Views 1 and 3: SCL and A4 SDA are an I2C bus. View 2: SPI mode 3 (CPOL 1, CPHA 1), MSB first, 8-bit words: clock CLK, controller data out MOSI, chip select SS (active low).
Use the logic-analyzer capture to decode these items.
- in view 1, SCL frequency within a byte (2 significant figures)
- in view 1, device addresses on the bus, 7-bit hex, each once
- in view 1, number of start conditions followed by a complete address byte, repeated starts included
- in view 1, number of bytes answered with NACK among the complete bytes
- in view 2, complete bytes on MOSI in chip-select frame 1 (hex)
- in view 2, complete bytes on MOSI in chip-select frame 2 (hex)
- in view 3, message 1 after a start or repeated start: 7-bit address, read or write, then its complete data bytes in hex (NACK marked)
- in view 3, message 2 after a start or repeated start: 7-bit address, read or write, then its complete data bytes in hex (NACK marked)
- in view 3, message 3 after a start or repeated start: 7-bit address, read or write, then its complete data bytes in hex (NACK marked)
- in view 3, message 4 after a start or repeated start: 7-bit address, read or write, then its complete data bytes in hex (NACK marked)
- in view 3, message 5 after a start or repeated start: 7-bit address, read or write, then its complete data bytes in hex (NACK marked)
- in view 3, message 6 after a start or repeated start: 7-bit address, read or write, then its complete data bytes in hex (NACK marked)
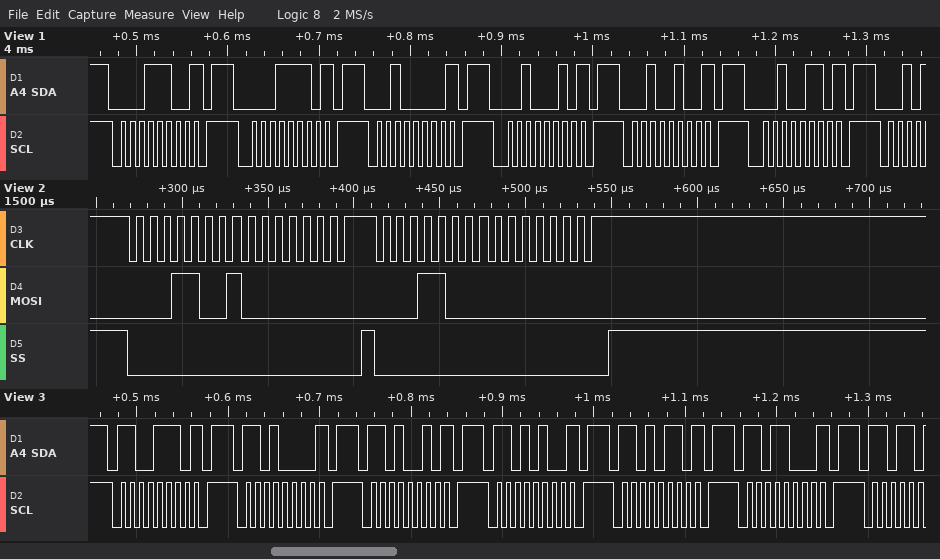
100 kHz
0x0E 0x0F 0x10 0x11 0x12 0x13
6
6
19 00
18 00
0x67 write NACK
0x68 write NACK
0x69 write NACK
0x6A write NACK
0x6B write NACK
0x6C write NACK
